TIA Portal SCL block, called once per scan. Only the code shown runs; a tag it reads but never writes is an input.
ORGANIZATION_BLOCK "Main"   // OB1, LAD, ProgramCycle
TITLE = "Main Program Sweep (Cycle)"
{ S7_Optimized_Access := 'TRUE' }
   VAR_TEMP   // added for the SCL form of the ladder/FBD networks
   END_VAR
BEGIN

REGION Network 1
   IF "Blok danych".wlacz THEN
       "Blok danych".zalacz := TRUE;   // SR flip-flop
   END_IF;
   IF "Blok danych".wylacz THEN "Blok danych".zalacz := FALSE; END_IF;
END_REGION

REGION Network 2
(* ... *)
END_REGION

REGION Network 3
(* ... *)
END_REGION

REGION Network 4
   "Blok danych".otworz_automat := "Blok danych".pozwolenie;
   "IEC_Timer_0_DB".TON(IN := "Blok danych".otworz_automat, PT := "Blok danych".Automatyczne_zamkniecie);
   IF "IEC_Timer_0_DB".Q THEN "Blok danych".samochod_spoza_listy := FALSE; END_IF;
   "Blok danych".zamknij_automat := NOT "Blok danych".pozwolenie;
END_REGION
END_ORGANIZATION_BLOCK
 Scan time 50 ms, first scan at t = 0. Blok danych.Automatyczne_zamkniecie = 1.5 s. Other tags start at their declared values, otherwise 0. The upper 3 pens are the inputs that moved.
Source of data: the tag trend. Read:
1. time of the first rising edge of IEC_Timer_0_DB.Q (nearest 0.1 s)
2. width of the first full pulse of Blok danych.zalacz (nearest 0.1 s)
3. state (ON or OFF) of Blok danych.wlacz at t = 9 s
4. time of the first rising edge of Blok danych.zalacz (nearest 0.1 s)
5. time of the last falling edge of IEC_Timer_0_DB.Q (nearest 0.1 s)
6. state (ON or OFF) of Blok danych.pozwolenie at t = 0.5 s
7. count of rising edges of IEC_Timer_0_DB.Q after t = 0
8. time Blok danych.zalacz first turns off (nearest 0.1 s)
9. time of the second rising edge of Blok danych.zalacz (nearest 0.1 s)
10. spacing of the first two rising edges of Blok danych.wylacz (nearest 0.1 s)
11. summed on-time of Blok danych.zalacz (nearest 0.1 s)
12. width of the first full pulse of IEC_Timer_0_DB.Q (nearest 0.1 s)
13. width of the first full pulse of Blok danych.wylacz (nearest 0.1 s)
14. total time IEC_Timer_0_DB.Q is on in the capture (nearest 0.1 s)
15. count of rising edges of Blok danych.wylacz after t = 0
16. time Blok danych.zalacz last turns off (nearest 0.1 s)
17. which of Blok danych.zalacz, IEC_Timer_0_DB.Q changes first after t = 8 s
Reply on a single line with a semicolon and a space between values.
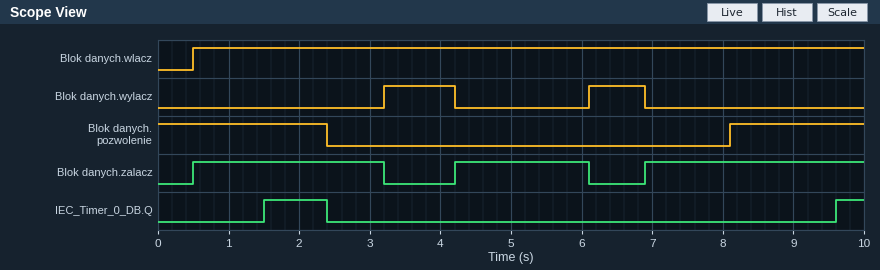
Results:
1.5 s; 2.7 s; ON; 0.5 s; 2.4 s; ON; 2; 3.2 s; 4.2 s; 2.9 s; 7.7 s; 0.9 s; 1.0 s; 1.3 s; 2; 6.1 s; IEC_Timer_0_DB.Q
